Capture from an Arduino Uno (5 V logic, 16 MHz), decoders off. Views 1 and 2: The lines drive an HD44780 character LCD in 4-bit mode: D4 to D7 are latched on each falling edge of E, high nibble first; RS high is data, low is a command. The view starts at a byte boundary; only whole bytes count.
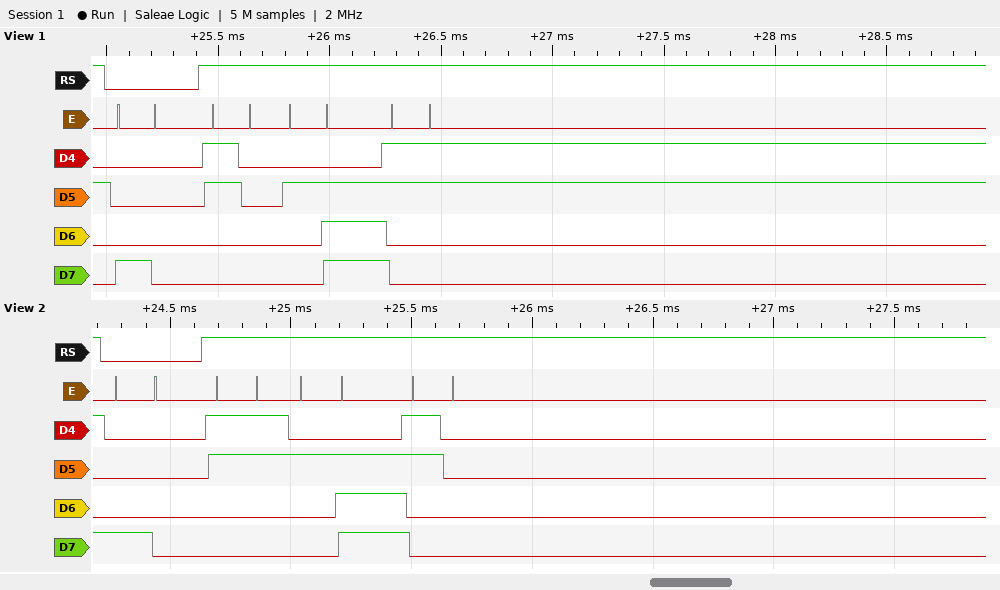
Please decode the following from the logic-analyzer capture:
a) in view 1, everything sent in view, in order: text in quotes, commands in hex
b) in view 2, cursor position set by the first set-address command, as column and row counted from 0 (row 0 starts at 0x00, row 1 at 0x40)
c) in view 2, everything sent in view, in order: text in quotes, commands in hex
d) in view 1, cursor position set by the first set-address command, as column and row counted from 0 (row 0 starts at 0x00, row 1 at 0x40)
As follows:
0x80 "0.3"
column 0, row 0
0x80 "3.0"
column 0, row 0
